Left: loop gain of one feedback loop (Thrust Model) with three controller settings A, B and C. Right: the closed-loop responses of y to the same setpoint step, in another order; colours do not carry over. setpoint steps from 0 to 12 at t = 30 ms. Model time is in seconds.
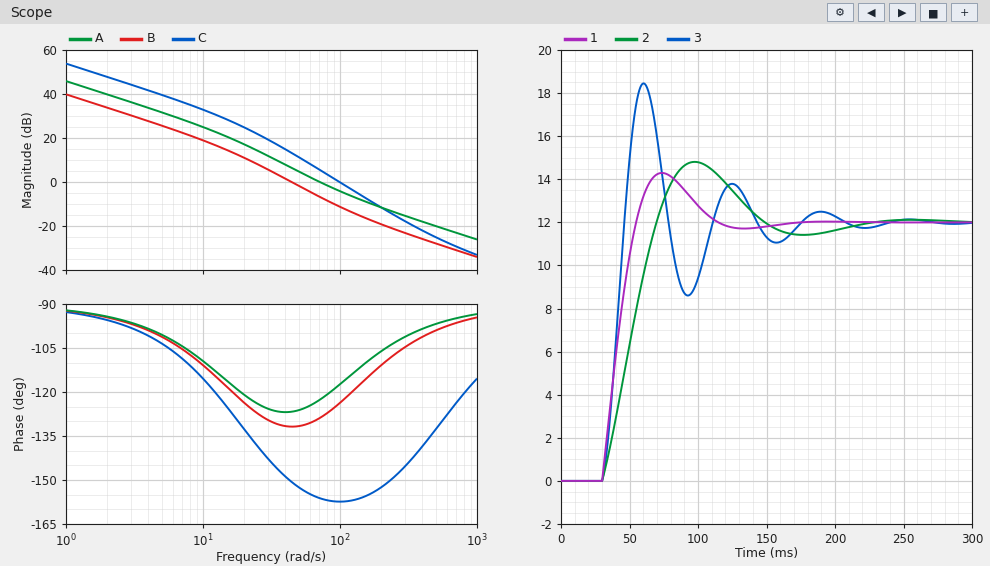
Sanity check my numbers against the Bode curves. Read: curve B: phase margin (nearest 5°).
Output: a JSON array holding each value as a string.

["50°"]
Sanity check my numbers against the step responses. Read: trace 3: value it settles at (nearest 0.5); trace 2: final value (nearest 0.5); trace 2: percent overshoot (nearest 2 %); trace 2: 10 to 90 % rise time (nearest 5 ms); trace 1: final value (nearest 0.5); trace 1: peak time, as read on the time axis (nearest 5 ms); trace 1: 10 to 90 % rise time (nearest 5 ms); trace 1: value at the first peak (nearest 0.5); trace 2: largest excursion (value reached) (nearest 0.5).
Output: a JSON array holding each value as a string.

["12.0", "12.0", "24 %", "30 ms", "12.0", "75 ms", "20 ms", "14.5", "15.0"]
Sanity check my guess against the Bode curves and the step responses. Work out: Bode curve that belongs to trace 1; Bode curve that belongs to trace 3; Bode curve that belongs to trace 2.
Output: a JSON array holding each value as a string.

["A", "C", "B"]
